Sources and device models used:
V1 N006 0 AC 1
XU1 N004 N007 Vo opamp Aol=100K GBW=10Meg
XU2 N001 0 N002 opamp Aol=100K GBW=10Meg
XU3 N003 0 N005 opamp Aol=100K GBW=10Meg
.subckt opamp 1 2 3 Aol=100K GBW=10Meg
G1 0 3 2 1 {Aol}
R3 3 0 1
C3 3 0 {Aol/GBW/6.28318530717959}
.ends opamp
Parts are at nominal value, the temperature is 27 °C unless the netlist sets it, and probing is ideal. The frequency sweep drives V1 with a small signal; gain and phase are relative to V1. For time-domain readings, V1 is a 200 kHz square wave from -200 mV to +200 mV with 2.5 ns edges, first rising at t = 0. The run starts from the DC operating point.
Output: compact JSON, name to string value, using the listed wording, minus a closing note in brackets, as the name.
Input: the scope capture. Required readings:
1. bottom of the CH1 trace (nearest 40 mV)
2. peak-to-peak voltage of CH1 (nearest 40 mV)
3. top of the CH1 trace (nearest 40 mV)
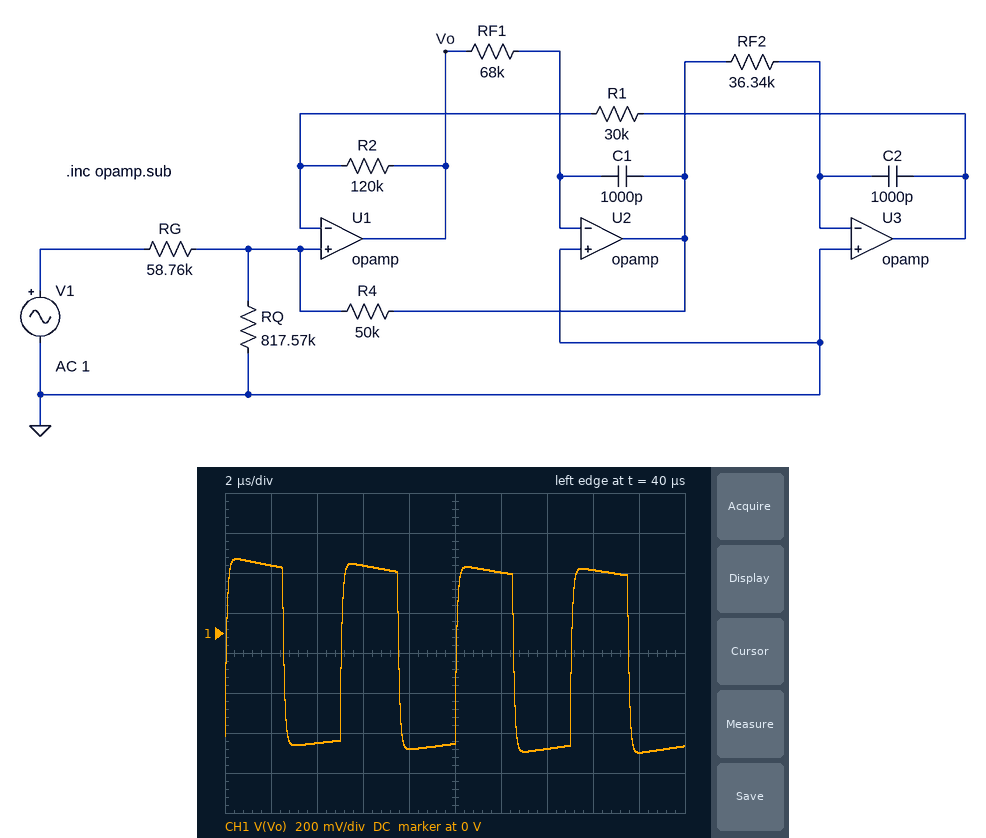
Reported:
{"bottom of the CH1 trace": "-600 mV", "peak-to-peak voltage of CH1": "960 mV", "top of the CH1 trace": "360 mV"}
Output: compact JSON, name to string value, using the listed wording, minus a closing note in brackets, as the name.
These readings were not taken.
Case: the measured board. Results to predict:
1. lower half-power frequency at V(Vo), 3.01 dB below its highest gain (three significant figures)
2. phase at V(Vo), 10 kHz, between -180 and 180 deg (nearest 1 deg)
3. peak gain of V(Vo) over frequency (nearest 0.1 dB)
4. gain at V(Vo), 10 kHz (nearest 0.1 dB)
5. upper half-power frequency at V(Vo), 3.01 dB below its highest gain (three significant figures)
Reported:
{"lower half-power frequency at V(Vo), 3.01 dB below its highest gain": "5.45 kHz", "phase at V(Vo), 10 kHz, between -180 and 180 deg": "46 deg", "peak gain of V(Vo) over frequency": "8.5 dB", "gain at V(Vo), 10 kHz": "8.4 dB", "upper half-power frequency at V(Vo), 3.01 dB below its highest gain": "1.27 MHz"}
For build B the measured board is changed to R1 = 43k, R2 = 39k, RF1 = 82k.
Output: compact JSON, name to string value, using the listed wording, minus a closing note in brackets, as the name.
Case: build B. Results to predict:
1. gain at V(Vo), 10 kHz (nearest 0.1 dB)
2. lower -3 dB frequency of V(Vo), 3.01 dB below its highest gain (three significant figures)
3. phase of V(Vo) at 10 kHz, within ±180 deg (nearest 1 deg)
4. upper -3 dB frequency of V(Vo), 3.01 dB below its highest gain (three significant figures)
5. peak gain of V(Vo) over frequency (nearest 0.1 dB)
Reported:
{"gain at V(Vo), 10 kHz": "-0.9 dB", "lower -3 dB frequency of V(Vo), 3.01 dB below its highest gain": "2.34 kHz", "phase of V(Vo) at 10 kHz, within ±180 deg": "12 deg", "upper -3 dB frequency of V(Vo), 3.01 dB below its highest gain": "8.58 kHz", "peak gain of V(Vo) over frequency": "2.3 dB"}
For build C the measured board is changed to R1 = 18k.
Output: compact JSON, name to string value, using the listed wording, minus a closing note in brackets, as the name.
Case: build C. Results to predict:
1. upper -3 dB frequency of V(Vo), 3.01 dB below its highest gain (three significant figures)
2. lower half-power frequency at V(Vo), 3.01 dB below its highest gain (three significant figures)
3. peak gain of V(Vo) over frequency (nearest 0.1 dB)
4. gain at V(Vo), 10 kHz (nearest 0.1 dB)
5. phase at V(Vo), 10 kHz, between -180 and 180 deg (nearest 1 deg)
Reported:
{"upper -3 dB frequency of V(Vo), 3.01 dB below its highest gain": "1.11 MHz", "lower half-power frequency at V(Vo), 3.01 dB below its highest gain": "7.30 kHz", "peak gain of V(Vo) over frequency": "11.3 dB", "gain at V(Vo), 10 kHz": "10.8 dB", "phase at V(Vo), 10 kHz, between -180 and 180 deg": "71 deg"}
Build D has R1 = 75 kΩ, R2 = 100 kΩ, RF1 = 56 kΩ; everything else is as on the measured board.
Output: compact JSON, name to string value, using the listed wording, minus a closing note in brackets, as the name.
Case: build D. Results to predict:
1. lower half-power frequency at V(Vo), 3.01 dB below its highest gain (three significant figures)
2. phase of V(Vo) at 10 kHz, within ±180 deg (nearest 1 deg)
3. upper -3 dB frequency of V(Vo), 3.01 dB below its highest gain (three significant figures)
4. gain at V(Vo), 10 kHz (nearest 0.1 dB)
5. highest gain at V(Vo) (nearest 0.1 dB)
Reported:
{"lower half-power frequency at V(Vo), 3.01 dB below its highest gain": "3.43 kHz", "phase of V(Vo) at 10 kHz, within ±180 deg": "22 deg", "upper -3 dB frequency of V(Vo), 3.01 dB below its highest gain": "1.84 MHz", "gain at V(Vo), 10 kHz": "1.2 dB", "highest gain at V(Vo)": "2.6 dB"}
